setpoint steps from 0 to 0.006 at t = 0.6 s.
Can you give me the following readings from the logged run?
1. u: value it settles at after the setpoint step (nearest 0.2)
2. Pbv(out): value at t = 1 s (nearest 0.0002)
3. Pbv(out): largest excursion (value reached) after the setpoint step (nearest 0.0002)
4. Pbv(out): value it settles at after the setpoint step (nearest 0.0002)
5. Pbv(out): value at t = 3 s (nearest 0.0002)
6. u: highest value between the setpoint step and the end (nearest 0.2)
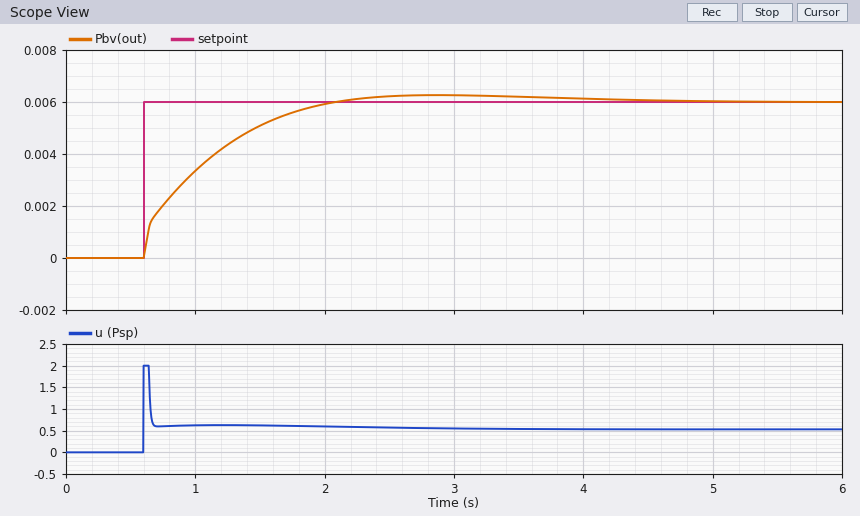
0.6
0.0034
0.0062
0.0060
0.0062
2.0
